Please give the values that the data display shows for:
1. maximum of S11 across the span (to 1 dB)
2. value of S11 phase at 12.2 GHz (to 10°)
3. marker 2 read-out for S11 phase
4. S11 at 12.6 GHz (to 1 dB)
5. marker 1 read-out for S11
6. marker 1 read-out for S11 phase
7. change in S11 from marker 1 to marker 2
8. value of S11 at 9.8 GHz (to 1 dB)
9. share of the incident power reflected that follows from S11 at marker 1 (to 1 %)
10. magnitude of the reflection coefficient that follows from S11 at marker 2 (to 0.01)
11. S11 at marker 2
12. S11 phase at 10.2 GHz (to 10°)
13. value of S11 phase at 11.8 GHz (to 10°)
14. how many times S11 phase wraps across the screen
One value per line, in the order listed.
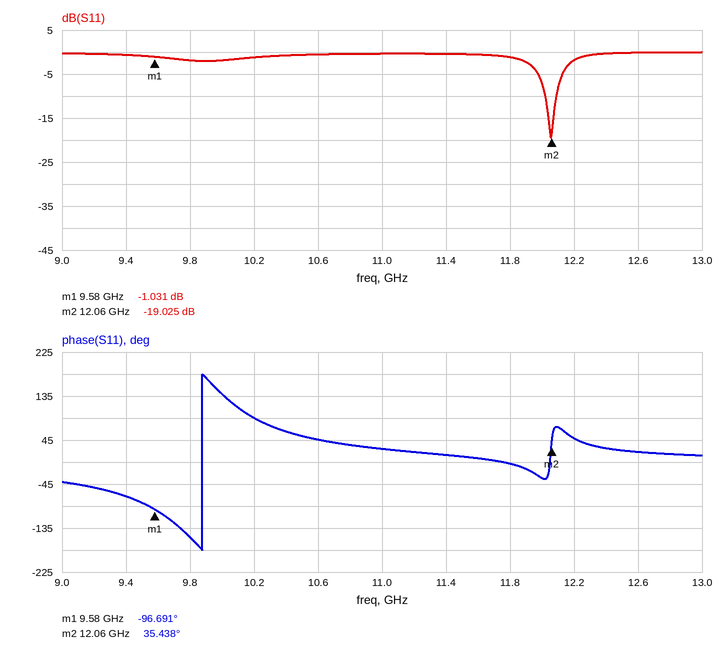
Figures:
0 dB
50°
35.438°
0 dB
-1.031 dB
-96.691°
-17.994 dB
-2 dB
79 %
0.11
-19.025 dB
90°
0°
1
